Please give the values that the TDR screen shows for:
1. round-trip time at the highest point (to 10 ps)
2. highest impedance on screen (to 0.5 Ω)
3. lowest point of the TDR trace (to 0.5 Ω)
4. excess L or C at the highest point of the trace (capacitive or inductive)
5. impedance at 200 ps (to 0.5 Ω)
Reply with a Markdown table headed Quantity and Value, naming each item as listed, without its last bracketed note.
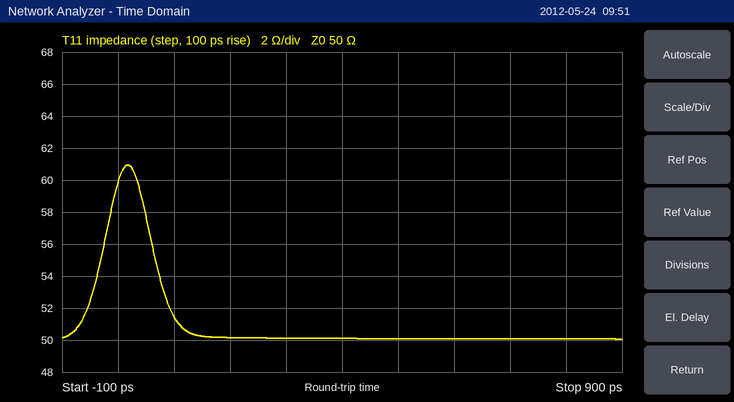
| Quantity | Value |
|---|---|
| round-trip time at the highest point | 20 ps |
| highest impedance on screen | 61.0 Ω |
| lowest point of the TDR trace | 50.0 Ω |
| excess L or C at the highest point of the trace | inductive |
| impedance at 200 ps | 50.0 Ω |
